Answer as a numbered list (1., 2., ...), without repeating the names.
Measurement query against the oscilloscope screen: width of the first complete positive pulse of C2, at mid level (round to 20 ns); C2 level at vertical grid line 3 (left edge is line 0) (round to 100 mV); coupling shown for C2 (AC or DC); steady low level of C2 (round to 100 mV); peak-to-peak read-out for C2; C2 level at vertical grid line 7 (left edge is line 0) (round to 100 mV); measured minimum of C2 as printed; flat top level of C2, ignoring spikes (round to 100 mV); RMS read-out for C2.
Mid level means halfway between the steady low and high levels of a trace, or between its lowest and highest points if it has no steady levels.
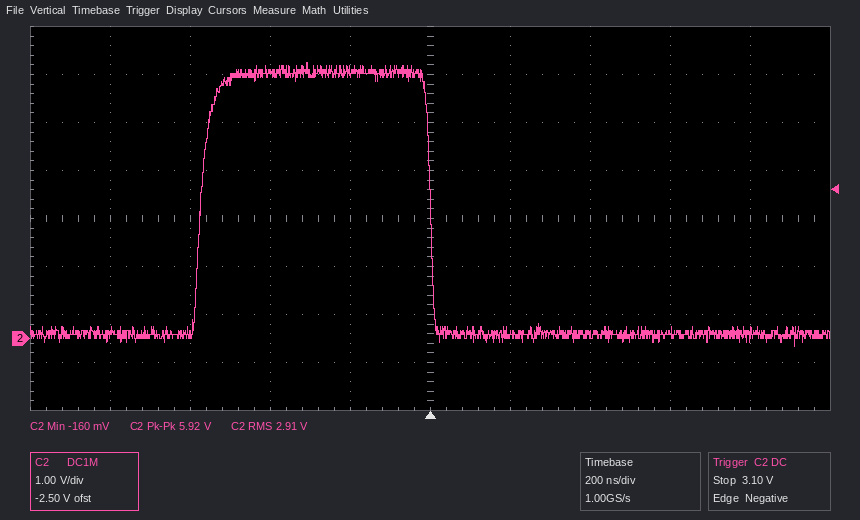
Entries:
1. 580 ns
2. 5.5 V
3. DC
4. 100 mV
5. 5.92 V
6. 100 mV
7. -160 mV
8. 5.5 V
9. 2.91 V
